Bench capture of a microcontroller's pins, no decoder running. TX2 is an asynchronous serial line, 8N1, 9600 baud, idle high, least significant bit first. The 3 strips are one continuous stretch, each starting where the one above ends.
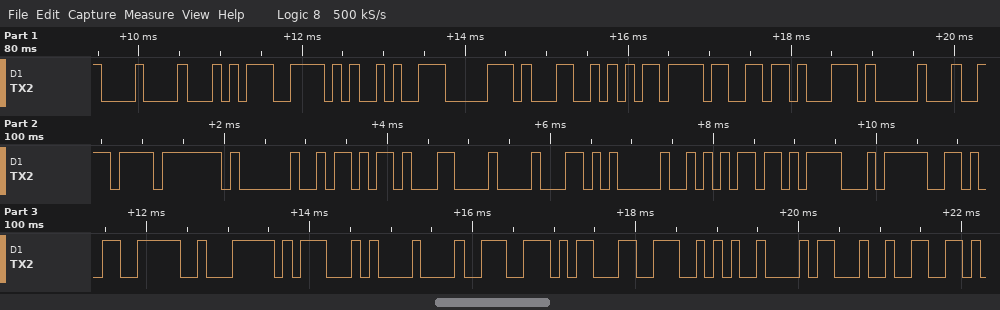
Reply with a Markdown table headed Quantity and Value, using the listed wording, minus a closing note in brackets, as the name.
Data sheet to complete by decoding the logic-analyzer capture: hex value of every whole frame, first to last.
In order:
| Quantity | Value |
|---|---|
| hex value of every whole frame, first to last | 0x08 0xD4 0x5E 0xCA 0x70 0x4C 0xED 0xB3 0x71 0x10 0xEE 0x7F 0x20 0x6B 0x0C 0x88 0x05 0xAA 0xEB 0xF4 0x96 0x3E 0x7C 0x47 0x08 0xCE 0x8D 0x4E 0x09 0x23 0x66 |
